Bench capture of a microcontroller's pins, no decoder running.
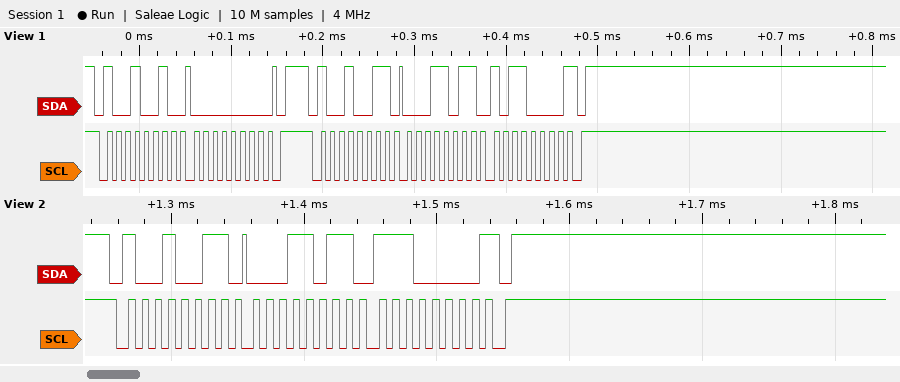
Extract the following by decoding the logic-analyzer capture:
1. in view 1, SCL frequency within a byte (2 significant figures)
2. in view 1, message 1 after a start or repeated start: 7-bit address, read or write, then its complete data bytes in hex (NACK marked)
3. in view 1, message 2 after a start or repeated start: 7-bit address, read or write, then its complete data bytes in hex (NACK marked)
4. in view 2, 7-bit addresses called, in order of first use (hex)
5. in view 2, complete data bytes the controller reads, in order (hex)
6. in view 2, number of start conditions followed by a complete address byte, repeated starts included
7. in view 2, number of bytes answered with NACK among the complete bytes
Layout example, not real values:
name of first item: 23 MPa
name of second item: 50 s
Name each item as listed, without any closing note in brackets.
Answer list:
in view 1, SCL frequency within a byte: 100 kHz
in view 1, message 1 after a start or repeated start: 7-bit address, read or write, then its complete data bytes in hex: 0x49 write: 00
in view 1, message 2 after a start or repeated start: 7-bit address, read or write, then its complete data bytes in hex: 0x49 read: 1B B0 NACK
in view 2, 7-bit addresses called, in order of first use: 0x49
in view 2, complete data bytes the controller reads, in order: 1B E0
in view 2, number of start conditions followed by a complete address byte, repeated starts included: 1
in view 2, number of bytes answered with NACK among the complete bytes: 1
